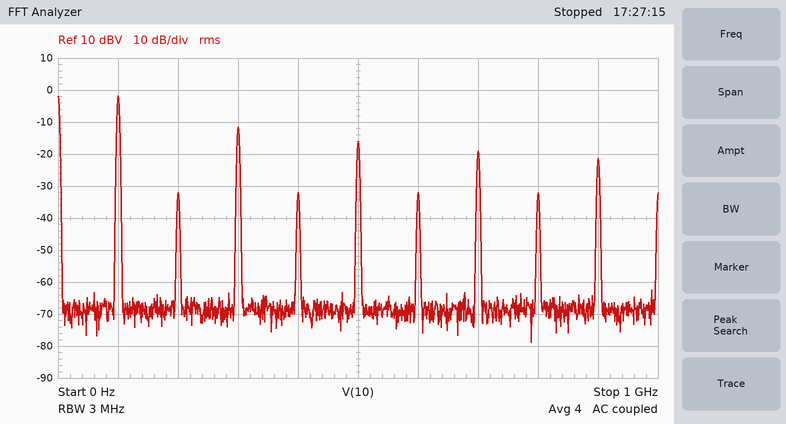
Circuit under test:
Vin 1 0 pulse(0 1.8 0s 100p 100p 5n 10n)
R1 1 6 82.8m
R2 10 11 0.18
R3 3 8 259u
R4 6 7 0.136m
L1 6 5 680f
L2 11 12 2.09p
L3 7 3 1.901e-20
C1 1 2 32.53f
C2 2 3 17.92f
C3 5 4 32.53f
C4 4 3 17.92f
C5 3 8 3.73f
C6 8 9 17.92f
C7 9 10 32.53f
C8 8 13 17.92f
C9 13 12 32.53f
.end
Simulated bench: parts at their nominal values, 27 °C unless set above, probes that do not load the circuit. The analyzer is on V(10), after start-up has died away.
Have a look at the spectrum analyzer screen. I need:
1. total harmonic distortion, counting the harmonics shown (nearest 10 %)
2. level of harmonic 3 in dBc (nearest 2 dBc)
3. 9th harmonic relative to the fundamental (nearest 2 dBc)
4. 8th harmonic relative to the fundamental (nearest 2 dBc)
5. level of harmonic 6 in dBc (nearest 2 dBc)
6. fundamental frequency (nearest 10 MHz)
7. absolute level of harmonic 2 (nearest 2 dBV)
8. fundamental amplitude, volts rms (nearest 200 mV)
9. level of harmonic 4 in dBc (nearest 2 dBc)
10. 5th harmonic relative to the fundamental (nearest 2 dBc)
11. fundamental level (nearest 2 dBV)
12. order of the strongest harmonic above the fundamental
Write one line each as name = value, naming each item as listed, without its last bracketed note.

total harmonic distortion, counting the harmonics shown = 40 %
level of harmonic 3 in dBc = -10 dBc
9th harmonic relative to the fundamental = -20 dBc
8th harmonic relative to the fundamental = -30 dBc
level of harmonic 6 in dBc = -30 dBc
fundamental frequency = 100 MHz
absolute level of harmonic 2 = -32 dBV
fundamental amplitude, volts rms = 800 mV
level of harmonic 4 in dBc = -30 dBc
5th harmonic relative to the fundamental = -14 dBc
fundamental level = -2 dBV
order of the strongest harmonic above the fundamental = 3
